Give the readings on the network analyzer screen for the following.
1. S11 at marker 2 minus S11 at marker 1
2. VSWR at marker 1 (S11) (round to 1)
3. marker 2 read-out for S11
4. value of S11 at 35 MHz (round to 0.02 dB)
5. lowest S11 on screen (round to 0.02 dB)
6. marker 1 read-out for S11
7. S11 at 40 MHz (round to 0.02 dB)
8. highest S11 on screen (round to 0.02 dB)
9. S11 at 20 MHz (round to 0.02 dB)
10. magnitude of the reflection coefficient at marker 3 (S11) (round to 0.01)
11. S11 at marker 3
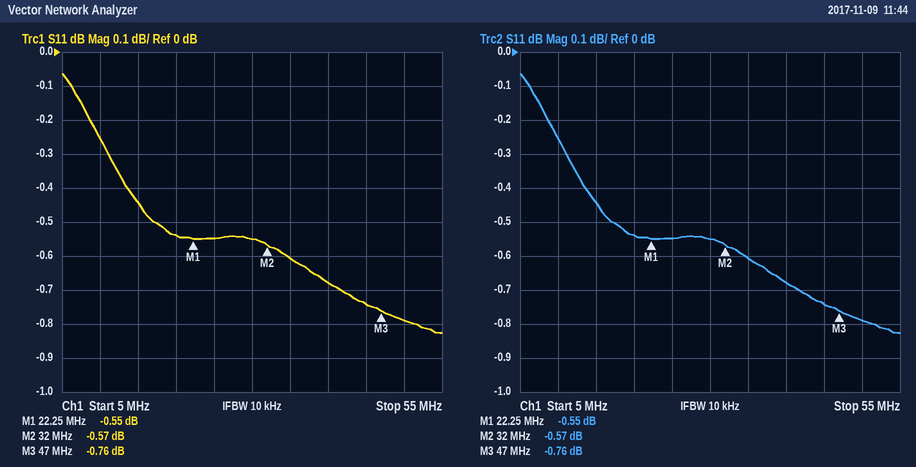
-0.02 dB
32
-0.57 dB
-0.60 dB
-0.82 dB
-0.55 dB
-0.68 dB
-0.06 dB
-0.54 dB
0.92
-0.76 dB
